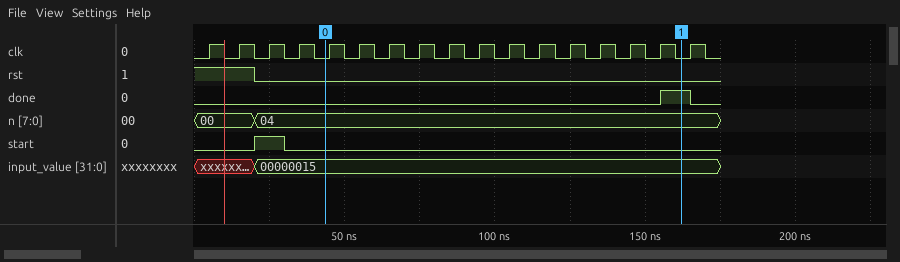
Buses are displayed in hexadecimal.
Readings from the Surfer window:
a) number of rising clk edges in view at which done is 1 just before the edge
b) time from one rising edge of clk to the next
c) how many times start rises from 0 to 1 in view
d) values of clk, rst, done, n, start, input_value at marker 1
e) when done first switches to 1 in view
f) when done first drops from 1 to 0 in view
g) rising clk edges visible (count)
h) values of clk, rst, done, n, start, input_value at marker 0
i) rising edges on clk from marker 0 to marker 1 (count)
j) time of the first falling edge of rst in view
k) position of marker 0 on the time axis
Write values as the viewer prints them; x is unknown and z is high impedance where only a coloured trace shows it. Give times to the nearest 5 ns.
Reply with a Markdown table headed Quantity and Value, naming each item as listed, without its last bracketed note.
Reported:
| Quantity | Value |
|---|---|
| number of rising clk edges in view at which done is 1 just before the edge | 1 |
| time from one rising edge of clk to the next | 10 ns |
| how many times start rises from 0 to 1 in view | 1 |
| values of clk, rst, done, n, start, input_value at marker 1 | clk=0, rst=0, done=1, n=04, start=0, input_value=00000015 |
| when done first switches to 1 in view | 155 ns |
| when done first drops from 1 to 0 in view | 165 ns |
| rising clk edges visible | 17 |
| values of clk, rst, done, n, start, input_value at marker 0 | clk=0, rst=0, done=0, n=04, start=0, input_value=00000015 |
| rising edges on clk from marker 0 to marker 1 | 12 |
| time of the first falling edge of rst in view | 20 ns |
| position of marker 0 on the time axis | 45 ns |
